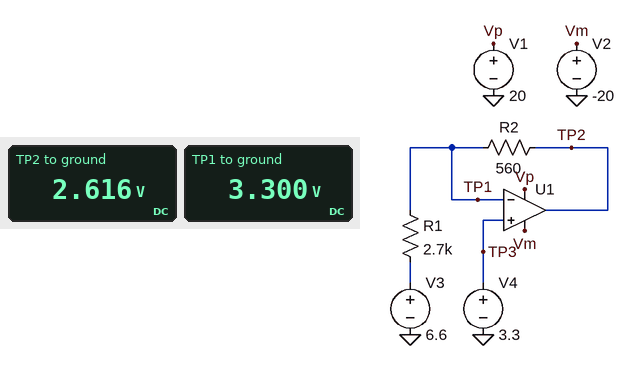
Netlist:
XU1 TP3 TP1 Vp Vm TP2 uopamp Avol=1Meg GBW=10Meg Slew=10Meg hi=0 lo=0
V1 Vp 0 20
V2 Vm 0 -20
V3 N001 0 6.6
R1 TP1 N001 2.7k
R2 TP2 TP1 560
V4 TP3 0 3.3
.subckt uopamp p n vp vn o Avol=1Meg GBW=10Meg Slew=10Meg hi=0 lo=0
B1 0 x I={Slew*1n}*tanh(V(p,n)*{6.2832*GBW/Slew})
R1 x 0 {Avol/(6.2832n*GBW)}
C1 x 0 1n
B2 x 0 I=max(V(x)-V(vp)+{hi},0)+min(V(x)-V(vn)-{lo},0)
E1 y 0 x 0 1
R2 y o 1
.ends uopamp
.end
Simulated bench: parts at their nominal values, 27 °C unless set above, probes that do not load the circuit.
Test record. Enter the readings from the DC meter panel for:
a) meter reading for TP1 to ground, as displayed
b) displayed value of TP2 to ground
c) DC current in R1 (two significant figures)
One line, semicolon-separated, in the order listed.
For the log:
3.300 V; 2.616 V; 1.2 mA
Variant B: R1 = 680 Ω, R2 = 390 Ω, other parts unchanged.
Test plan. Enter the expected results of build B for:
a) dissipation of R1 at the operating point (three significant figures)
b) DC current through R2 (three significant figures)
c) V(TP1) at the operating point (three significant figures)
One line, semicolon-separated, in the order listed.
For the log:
16.0 mW; 4.85 mA; 3.30 V
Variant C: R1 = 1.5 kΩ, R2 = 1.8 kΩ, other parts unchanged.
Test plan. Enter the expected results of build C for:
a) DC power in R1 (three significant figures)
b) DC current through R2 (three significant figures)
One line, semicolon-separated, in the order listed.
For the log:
7.26 mW; 2.20 mA
